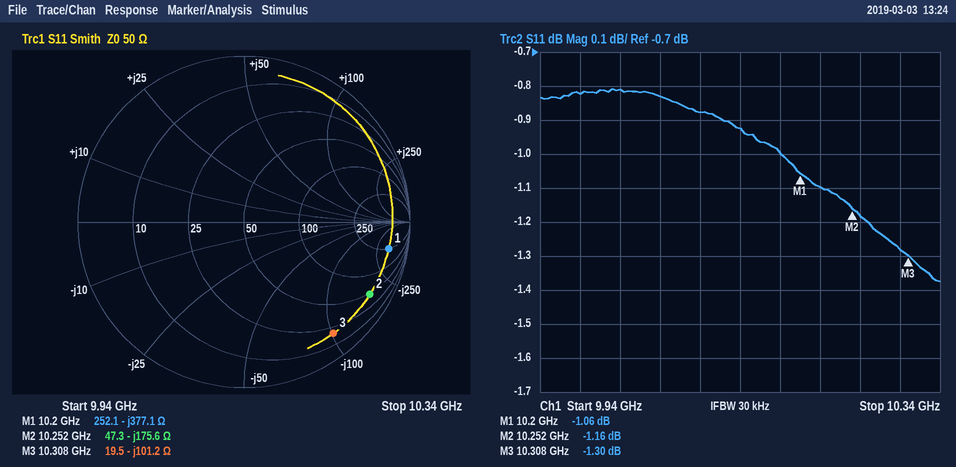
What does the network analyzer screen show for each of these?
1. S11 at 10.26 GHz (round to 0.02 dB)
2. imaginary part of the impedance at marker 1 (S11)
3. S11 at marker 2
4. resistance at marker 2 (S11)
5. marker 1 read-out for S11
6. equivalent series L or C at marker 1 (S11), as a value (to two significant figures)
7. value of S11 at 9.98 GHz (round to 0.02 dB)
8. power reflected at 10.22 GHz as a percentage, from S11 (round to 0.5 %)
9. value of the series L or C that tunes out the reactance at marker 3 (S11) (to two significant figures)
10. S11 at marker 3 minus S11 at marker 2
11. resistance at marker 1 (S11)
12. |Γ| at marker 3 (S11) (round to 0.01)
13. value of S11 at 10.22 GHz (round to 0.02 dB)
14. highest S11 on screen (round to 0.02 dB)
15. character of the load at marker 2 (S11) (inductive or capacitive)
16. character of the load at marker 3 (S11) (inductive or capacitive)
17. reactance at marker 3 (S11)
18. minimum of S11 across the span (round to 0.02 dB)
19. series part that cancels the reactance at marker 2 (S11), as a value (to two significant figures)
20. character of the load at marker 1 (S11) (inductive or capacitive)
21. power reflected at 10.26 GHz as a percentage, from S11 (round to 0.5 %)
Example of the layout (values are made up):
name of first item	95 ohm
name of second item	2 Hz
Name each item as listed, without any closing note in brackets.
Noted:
S11 at 10.26 GHz	-1.18 dB
imaginary part of the impedance at marker 1	-377.1 Ω
S11 at marker 2	-1.16 dB
resistance at marker 2	47.3 Ω
marker 1 read-out for S11	-1.06 dB
equivalent series L or C at marker 1 (S11), as a value	41 fF
value of S11 at 9.98 GHz	-0.82 dB
power reflected at 10.22 GHz as a percentage, from S11	77.5 %
value of the series L or C that tunes out the reactance at marker 3 (S11)	1.6 nH
S11 at marker 3 minus S11 at marker 2	-0.14 dB
resistance at marker 1	252.1 Ω
|Γ| at marker 3 (S11)	0.86
value of S11 at 10.22 GHz	-1.10 dB
highest S11 on screen	-0.80 dB
character of the load at marker 2 (S11)	capacitive
character of the load at marker 3 (S11)	capacitive
reactance at marker 3	-101.2 Ω
minimum of S11 across the span	-1.38 dB
series part that cancels the reactance at marker 2 (S11), as a value	2.7 nH
character of the load at marker 1 (S11)	capacitive
power reflected at 10.26 GHz as a percentage, from S11	76.0 %
